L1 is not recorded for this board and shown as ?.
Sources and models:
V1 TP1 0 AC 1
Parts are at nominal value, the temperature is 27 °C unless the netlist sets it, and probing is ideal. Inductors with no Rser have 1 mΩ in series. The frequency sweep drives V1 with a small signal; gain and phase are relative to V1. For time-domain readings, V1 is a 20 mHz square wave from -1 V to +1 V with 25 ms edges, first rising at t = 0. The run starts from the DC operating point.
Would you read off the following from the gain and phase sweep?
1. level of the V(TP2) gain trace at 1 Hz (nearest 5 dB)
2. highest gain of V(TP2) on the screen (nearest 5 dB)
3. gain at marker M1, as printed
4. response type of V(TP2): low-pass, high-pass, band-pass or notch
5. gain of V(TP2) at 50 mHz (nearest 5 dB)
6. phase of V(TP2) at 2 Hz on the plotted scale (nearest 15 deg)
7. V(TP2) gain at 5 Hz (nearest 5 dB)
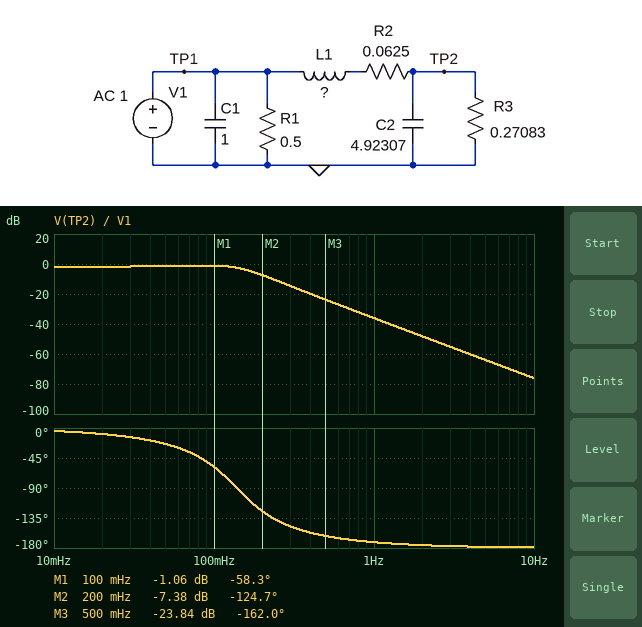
-35 dB
0 dB
-1.06 dB
low-pass
0 dB
-180 deg
-65 dB
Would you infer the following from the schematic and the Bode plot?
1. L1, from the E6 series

330 mH
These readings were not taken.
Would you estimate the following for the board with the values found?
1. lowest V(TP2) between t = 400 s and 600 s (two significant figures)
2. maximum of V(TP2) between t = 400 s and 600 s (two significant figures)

-1.0 V
1.0 V
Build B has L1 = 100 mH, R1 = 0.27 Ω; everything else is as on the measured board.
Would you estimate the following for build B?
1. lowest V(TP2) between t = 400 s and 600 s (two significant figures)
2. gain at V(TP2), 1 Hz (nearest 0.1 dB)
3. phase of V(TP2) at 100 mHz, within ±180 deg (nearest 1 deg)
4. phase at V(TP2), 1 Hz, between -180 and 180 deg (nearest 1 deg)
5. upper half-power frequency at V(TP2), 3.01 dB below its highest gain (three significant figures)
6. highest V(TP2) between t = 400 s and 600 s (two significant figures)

-1.2 V
-25.4 dB
-22 deg
-167 deg
299 mHz
1.2 V
